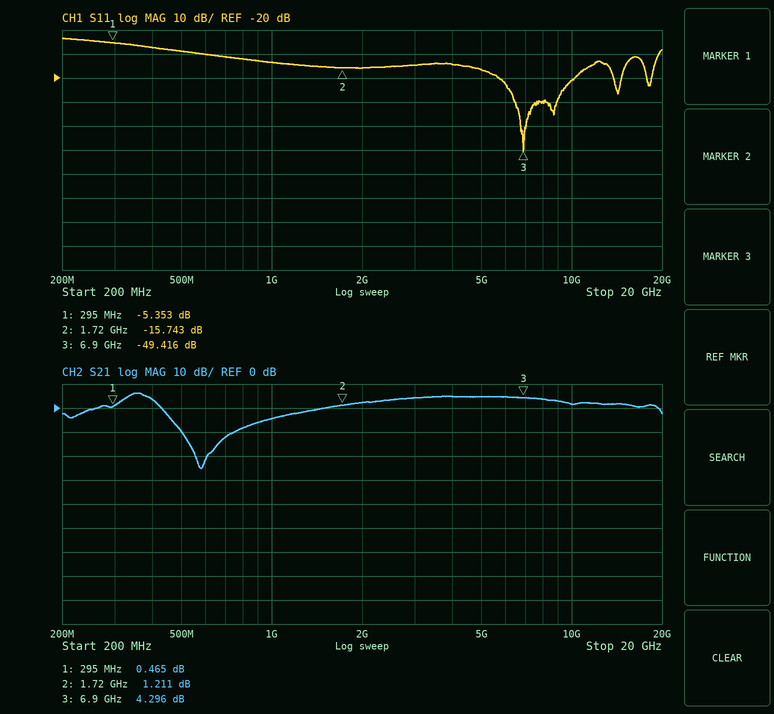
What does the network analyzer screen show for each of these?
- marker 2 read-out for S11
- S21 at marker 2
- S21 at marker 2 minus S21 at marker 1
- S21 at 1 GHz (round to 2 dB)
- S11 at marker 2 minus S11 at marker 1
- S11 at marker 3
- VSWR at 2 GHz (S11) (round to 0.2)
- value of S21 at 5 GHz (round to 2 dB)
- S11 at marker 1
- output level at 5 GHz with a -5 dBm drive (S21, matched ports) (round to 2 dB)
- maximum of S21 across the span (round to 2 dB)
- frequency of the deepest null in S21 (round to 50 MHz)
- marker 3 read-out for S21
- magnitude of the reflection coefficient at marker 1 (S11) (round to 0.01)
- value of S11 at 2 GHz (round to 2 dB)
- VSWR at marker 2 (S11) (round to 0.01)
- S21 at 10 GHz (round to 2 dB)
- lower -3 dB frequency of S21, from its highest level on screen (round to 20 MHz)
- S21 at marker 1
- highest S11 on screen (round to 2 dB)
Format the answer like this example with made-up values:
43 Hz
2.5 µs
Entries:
-15.743 dB
1.211 dB
0.746 dB
-4 dB
-10.390 dB
-49.416 dB
1.4
4 dB
-5.353 dB
0 dBm
6 dB
600 MHz
4.296 dB
0.54
-16 dB
1.39
2 dB
320 MHz
0.465 dB
-4 dB
